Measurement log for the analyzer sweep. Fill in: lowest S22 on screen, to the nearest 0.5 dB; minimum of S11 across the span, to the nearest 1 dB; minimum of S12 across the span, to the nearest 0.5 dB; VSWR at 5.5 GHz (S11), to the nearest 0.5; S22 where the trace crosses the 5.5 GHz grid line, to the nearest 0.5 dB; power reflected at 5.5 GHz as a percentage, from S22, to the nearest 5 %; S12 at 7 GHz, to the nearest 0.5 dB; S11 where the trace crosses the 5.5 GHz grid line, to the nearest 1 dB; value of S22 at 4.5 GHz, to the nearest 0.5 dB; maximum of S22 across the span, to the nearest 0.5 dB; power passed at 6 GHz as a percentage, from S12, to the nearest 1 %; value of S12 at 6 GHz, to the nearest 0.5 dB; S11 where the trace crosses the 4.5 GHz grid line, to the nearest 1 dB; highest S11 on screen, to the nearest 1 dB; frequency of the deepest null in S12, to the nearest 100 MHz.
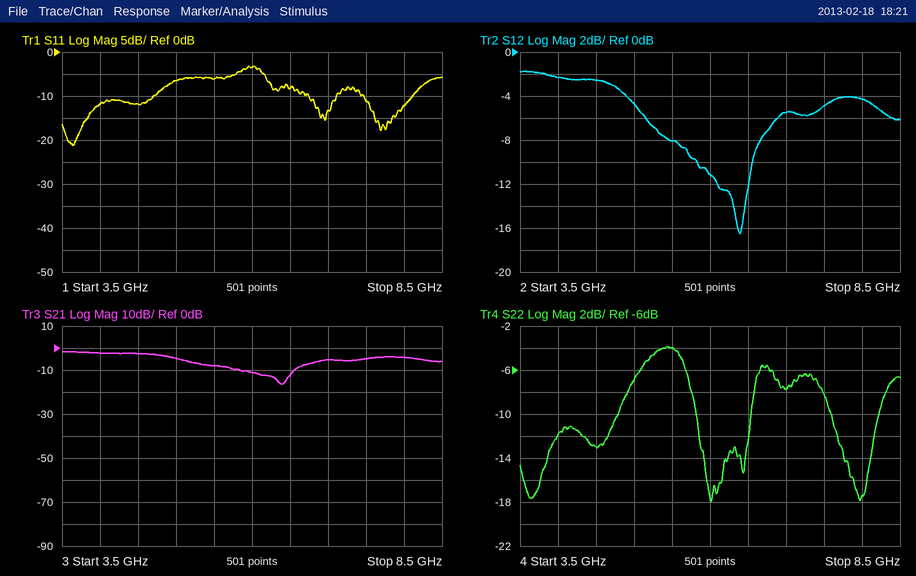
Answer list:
-18.0 dB
-21 dB
-16.5 dB
3.0
-4.0 dB
40 %
-5.5 dB
-6 dB
-13.0 dB
-4.0 dB
8 %
-11.0 dB
-12 dB
-3 dB
6.4 GHz
